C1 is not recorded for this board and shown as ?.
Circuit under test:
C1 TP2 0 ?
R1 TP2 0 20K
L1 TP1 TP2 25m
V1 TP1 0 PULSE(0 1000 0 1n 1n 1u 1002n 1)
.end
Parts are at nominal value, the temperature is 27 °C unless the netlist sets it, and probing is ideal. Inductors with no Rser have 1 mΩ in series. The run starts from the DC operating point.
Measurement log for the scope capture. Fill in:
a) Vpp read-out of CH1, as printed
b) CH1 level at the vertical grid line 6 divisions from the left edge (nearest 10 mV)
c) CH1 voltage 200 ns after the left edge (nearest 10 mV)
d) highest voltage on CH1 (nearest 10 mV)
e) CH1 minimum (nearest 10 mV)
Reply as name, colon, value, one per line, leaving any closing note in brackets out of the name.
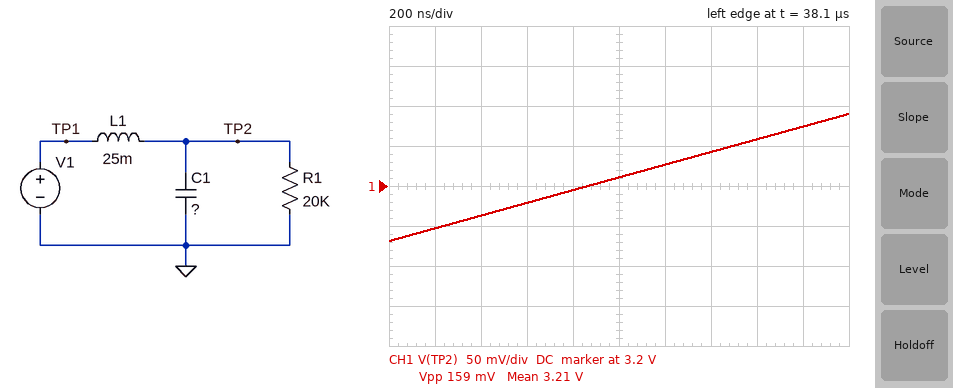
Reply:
Vpp read-out of CH1, as printed: 159 mV
CH1 level at the vertical grid line 6 divisions from the left edge: 3.23 V
CH1 voltage 200 ns after the left edge: 3.15 V
highest voltage on CH1: 3.29 V
CH1 minimum: 3.13 V
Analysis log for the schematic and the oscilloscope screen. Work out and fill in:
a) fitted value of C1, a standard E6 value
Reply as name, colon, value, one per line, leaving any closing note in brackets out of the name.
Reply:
fitted value of C1, a standard E6 value: 470 nF
